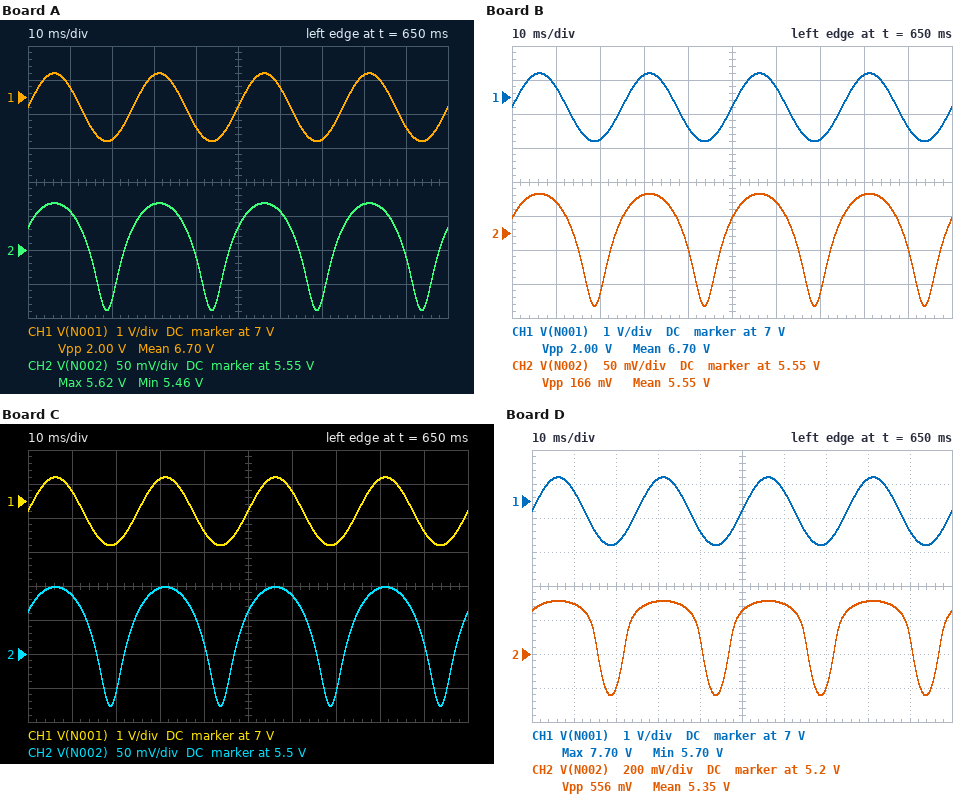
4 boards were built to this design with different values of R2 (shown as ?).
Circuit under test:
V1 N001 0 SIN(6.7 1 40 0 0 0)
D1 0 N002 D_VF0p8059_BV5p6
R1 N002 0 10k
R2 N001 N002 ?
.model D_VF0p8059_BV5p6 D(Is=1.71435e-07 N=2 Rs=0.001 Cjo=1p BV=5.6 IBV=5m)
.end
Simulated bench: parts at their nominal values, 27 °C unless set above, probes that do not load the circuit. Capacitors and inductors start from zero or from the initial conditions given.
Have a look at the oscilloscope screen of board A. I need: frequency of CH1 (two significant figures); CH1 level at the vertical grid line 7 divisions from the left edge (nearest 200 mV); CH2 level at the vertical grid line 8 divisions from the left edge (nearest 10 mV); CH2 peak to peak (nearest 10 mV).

40 Hz
5.8 V
5.62 V
160 mV
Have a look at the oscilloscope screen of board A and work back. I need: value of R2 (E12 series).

270 Ω
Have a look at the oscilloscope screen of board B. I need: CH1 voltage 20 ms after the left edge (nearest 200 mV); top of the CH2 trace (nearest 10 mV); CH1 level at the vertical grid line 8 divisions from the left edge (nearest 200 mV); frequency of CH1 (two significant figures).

5.8 V
5.61 V
7.6 V
40 Hz
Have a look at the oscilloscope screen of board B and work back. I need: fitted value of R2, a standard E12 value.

330 Ω
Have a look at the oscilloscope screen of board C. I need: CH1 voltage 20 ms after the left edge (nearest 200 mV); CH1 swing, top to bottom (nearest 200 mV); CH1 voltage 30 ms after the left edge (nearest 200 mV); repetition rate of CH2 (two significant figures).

5.8 V
2.0 V
7.6 V
40 Hz
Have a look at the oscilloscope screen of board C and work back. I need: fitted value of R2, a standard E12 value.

390 Ω
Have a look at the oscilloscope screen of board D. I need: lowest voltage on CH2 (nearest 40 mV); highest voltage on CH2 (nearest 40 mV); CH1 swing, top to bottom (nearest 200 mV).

4.96 V
5.52 V
2.0 V
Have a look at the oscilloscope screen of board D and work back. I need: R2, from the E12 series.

1.5 kΩ
